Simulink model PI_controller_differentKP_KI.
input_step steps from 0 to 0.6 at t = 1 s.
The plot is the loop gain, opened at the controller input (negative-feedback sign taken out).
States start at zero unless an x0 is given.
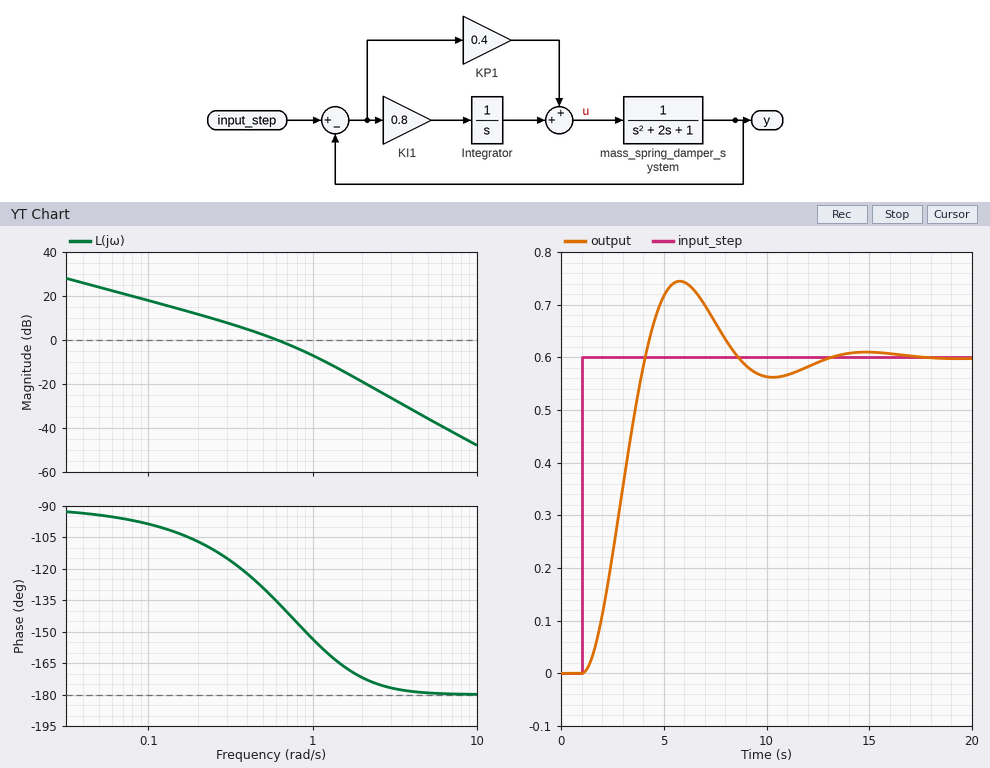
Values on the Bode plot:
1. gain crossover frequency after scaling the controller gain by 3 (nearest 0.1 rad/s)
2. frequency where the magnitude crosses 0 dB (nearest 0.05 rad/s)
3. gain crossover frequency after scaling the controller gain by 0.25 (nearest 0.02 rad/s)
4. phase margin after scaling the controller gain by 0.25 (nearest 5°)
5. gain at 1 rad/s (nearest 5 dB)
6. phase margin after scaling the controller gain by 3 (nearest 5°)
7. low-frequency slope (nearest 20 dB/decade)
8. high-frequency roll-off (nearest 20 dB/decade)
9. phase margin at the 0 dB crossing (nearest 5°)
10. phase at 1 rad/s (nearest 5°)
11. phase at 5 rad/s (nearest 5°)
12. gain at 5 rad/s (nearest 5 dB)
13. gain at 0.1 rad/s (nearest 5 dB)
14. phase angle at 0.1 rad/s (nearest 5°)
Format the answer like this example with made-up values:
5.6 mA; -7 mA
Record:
1.2 rad/s; 0.60 rad/s; 0.20 rad/s; 75°; -5 dB; 20°; -20 dB/decade; -40 dB/decade; 45°; -155°; -180°; -35 dB; 20 dB; -100°
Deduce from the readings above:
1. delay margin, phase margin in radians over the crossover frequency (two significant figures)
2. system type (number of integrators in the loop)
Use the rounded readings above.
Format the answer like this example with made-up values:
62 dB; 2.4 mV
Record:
1.3 s; 1
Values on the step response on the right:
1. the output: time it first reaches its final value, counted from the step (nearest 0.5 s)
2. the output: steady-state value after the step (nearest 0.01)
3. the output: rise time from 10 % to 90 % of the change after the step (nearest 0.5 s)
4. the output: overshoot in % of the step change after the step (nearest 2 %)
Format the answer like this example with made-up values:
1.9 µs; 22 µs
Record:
3.0 s; 0.60; 2.0 s; 24 %
